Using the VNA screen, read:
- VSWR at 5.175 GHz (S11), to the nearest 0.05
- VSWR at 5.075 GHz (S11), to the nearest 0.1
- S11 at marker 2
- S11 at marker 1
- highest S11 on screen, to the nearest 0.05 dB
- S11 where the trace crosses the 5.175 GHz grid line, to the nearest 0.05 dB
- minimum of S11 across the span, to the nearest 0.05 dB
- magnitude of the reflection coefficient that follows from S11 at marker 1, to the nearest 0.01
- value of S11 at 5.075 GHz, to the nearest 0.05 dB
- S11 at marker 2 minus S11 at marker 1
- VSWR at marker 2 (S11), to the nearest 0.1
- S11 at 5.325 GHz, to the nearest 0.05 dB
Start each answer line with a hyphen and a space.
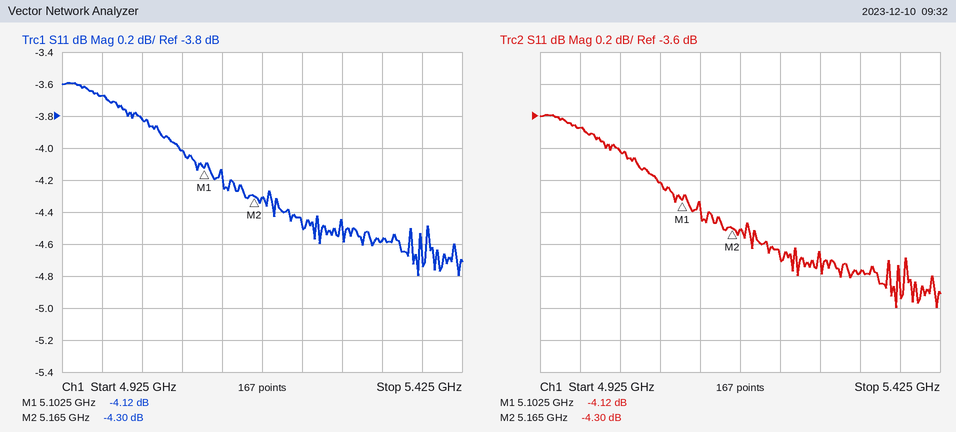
- 4.10
- 4.4
- -4.30 dB
- -4.12 dB
- -3.60 dB
- -4.30 dB
- -4.80 dB
- 0.62
- -4.00 dB
- -0.18 dB
- 4.1
- -4.60 dB
